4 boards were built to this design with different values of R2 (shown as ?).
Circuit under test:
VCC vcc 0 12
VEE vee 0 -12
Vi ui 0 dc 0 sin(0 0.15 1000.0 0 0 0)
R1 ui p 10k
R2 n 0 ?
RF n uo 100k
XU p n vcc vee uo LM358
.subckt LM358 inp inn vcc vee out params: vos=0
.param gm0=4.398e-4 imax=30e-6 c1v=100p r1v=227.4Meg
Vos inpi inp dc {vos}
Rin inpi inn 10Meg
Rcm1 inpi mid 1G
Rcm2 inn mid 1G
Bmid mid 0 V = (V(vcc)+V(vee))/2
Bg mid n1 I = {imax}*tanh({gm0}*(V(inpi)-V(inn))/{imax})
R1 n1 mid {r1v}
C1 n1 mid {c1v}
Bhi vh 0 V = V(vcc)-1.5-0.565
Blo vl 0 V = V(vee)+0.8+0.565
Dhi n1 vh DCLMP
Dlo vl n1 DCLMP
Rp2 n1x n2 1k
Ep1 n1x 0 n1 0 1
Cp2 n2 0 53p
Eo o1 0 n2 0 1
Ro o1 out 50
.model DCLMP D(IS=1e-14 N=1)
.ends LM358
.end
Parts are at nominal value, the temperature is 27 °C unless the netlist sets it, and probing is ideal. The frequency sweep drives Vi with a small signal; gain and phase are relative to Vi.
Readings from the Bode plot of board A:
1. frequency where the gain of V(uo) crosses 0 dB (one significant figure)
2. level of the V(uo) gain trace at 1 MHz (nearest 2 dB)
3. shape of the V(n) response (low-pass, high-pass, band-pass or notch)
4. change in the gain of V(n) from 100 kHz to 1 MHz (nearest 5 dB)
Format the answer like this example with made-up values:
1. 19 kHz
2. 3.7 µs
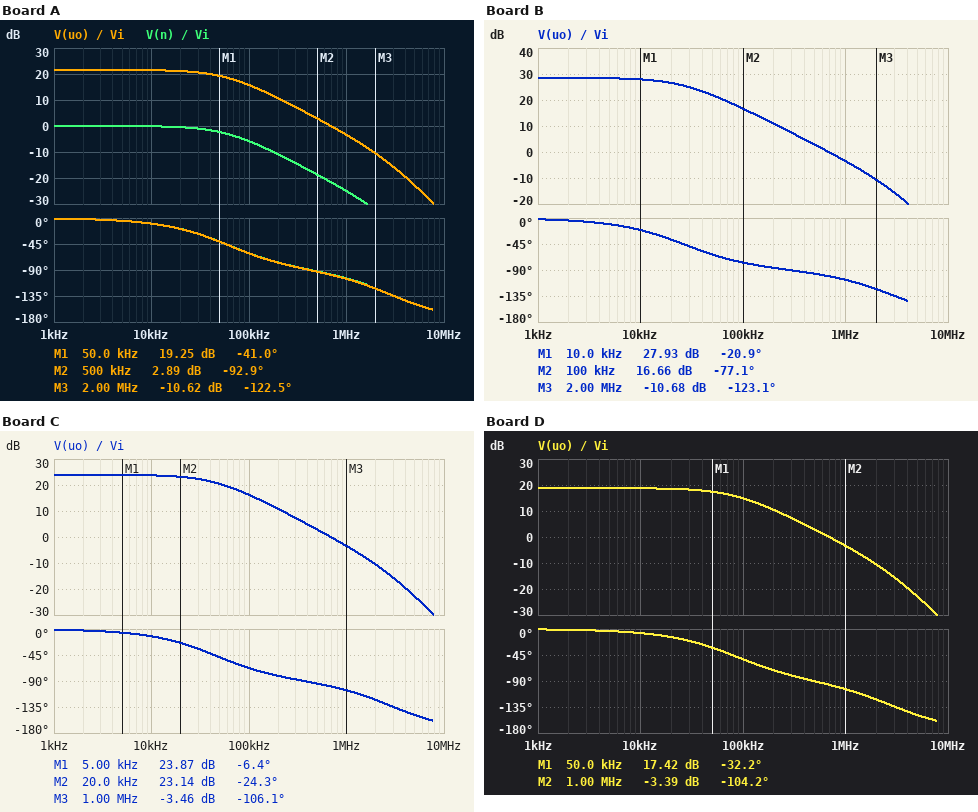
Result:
1. 700 kHz
2. -4 dB
3. low-pass
4. -20 dB
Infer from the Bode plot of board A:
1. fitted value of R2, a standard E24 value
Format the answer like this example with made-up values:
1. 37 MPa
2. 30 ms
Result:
1. 9.1 kΩ
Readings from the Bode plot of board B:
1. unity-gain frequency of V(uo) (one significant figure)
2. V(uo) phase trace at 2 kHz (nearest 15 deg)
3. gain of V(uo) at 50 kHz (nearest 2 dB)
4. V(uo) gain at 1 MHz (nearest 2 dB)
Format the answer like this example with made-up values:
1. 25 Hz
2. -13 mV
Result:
1. 700 kHz
2. 0 deg
3. 22 dB
4. -4 dB
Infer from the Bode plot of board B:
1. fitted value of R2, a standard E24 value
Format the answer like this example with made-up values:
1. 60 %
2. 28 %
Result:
1. 3.9 kΩ
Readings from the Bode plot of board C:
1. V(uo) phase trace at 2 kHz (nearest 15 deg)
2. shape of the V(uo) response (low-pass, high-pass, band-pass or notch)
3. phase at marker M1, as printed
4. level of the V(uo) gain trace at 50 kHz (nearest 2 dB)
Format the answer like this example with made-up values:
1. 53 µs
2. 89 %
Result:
1. 0 deg
2. low-pass
3. -6.4 deg
4. 20 dB
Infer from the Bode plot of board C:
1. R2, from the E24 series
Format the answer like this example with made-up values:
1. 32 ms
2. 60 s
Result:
1. 6.8 kΩ
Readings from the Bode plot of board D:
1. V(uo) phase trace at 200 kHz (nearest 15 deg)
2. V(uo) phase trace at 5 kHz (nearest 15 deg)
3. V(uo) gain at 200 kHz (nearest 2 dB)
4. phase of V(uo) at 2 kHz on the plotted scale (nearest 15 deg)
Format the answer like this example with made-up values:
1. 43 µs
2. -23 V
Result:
1. -75 deg
2. 0 deg
3. 10 dB
4. 0 deg
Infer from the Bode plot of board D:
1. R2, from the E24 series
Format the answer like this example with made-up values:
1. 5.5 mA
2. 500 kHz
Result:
1. 13 kΩ
